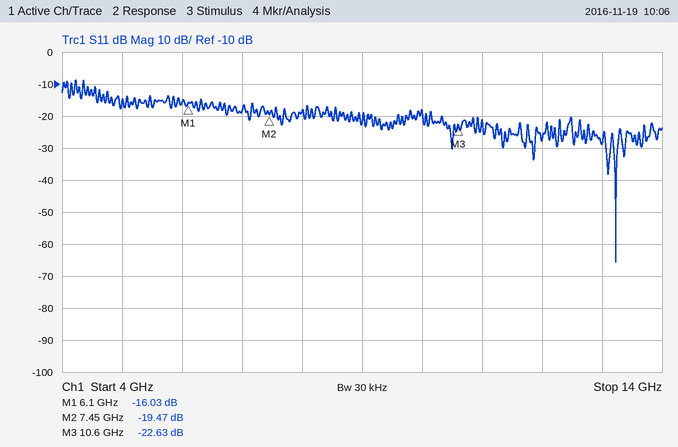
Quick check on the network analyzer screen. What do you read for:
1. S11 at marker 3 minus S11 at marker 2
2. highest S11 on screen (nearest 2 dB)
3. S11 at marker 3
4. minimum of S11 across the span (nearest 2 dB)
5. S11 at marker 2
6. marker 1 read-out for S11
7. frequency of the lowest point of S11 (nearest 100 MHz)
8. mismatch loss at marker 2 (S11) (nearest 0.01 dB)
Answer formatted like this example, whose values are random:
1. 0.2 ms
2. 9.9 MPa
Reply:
1. -3.16 dB
2. -8 dB
3. -22.63 dB
4. -66 dB
5. -19.47 dB
6. -16.03 dB
7. 13.2 GHz
8. 0.05 dB
